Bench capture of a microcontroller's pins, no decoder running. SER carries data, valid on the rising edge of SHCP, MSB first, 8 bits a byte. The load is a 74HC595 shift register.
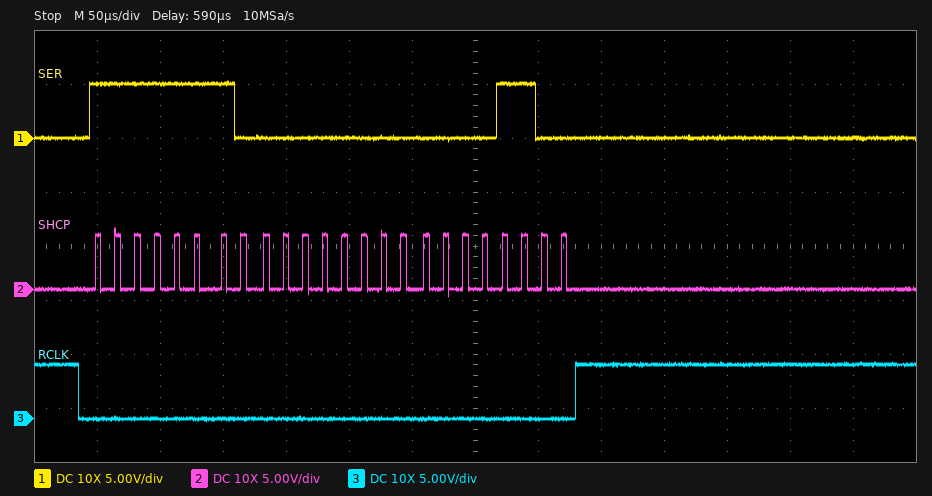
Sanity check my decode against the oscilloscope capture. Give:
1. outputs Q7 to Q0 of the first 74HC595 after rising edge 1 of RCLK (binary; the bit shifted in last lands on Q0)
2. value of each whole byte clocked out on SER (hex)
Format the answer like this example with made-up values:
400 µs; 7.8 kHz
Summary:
00001100; FE 00 0C
